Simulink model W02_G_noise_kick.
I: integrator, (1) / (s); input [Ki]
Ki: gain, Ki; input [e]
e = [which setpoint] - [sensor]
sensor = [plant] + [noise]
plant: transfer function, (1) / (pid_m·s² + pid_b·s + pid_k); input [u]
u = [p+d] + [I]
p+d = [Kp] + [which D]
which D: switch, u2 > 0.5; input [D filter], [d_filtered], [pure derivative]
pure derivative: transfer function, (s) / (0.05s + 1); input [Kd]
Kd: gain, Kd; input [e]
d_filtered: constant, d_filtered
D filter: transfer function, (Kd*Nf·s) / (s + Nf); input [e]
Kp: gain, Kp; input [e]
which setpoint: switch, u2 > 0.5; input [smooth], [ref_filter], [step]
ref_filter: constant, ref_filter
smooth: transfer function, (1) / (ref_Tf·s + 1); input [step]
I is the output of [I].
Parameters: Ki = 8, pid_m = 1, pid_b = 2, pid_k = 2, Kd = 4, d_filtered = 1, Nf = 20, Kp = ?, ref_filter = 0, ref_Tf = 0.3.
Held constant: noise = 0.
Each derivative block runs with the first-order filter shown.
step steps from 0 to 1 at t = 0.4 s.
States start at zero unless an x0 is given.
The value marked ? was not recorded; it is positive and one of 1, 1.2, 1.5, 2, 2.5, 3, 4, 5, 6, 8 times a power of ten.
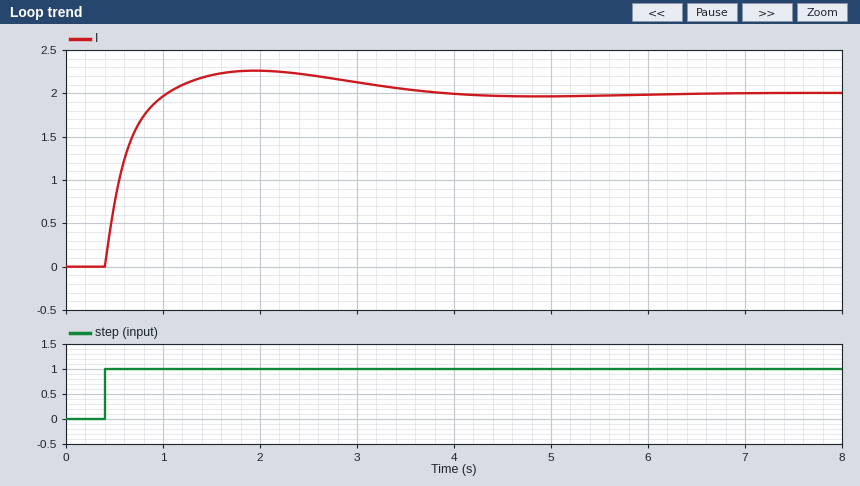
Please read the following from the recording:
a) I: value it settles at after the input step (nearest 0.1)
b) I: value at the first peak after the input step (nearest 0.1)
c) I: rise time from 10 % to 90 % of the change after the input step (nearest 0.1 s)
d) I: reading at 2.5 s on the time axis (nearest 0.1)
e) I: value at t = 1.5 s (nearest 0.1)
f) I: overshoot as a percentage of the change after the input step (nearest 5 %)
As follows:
2.0
2.3
0.4 s
2.2
2.2
15 %
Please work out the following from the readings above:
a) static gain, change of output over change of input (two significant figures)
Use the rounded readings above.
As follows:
2.0
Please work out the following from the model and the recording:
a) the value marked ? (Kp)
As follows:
6
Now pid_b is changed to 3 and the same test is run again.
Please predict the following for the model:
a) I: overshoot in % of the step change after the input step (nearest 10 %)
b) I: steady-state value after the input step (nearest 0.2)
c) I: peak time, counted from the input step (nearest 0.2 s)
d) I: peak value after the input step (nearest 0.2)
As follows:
40 %
2.0
1.6 s
2.8
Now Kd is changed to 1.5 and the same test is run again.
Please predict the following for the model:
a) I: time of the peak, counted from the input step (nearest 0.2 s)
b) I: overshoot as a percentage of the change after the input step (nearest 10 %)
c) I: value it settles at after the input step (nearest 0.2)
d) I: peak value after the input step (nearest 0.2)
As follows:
0.8 s
40 %
2.0
2.8
